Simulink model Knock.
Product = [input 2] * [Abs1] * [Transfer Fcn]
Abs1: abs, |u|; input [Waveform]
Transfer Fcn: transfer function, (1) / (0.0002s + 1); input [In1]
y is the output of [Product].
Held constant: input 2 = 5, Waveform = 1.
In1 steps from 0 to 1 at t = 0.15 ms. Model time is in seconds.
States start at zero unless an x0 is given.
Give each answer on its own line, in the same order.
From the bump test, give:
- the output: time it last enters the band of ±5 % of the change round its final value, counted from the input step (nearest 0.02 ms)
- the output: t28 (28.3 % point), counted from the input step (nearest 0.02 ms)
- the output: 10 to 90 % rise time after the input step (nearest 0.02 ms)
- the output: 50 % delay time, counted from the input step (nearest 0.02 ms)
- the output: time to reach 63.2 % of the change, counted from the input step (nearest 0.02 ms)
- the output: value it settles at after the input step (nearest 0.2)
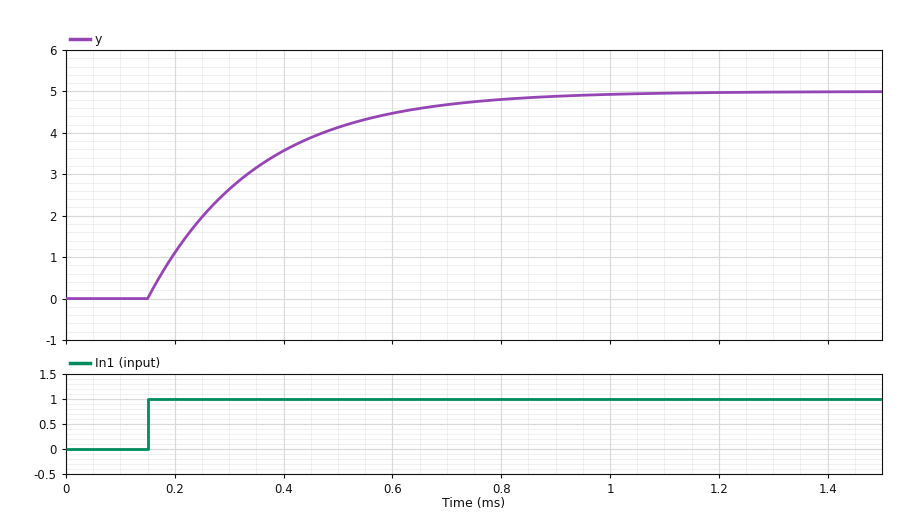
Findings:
0.60 ms
0.06 ms
0.44 ms
0.14 ms
0.20 ms
5.0
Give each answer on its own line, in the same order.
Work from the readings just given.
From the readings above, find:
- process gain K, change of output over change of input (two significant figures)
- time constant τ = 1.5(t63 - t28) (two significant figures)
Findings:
5.0
0.21 ms
